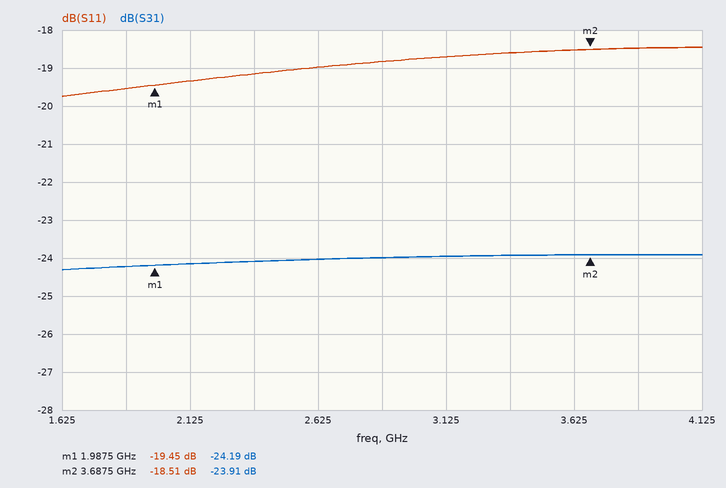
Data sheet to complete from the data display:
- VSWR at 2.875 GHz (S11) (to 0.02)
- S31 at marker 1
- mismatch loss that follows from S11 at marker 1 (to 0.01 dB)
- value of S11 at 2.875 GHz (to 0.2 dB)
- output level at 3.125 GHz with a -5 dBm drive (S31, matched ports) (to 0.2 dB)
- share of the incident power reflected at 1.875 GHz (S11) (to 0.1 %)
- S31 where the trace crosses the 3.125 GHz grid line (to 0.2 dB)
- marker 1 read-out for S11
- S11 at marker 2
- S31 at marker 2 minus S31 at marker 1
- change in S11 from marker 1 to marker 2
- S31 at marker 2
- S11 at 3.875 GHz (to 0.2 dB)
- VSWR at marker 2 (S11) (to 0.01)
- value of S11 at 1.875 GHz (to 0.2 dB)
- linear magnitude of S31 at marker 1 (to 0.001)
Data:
1.26
-24.19 dB
0.05 dB
-18.8 dB
-29.0 dBm
1.1 %
-24.0 dB
-19.45 dB
-18.51 dB
0.28 dB
0.94 dB
-23.91 dB
-18.4 dB
1.27
-19.6 dB
0.062
